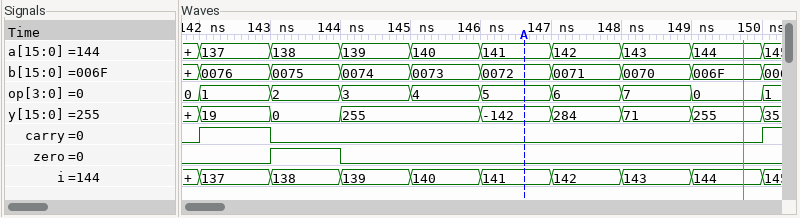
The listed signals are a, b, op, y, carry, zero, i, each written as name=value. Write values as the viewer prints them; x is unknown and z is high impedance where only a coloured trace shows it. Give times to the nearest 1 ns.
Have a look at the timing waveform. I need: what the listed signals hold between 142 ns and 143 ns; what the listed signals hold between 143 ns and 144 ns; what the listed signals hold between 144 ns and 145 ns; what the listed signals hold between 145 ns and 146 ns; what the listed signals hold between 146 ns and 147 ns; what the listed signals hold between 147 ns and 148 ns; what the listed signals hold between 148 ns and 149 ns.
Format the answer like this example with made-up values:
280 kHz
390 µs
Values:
a=137, b=0076, op=1, y=19, carry=1, zero=0, i=137
a=138, b=0075, op=2, y=0, carry=0, zero=1, i=138
a=139, b=0074, op=3, y=255, carry=0, zero=0, i=139
a=140, b=0073, op=4, y=255, carry=0, zero=0, i=140
a=141, b=0072, op=5, y=-142, carry=0, zero=0, i=141
a=142, b=0071, op=6, y=284, carry=0, zero=0, i=142
a=143, b=0070, op=7, y=71, carry=0, zero=0, i=143
